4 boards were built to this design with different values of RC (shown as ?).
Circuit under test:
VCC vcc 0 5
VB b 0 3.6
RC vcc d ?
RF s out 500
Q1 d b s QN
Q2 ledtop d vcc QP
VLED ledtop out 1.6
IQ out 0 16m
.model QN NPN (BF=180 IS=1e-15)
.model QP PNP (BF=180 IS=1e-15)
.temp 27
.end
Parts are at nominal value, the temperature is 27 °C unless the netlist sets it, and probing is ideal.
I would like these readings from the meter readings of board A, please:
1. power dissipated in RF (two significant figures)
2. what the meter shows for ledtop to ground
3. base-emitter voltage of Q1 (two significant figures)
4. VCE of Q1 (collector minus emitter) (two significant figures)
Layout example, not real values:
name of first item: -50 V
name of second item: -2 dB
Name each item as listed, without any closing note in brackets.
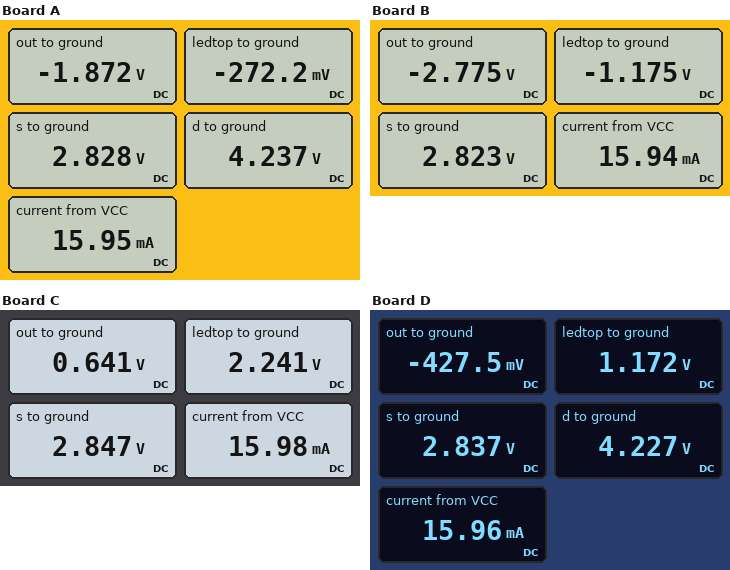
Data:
power dissipated in RF: 44 mW
what the meter shows for ledtop to ground: -272.2 mV
base-emitter voltage of Q1: 770 mV
VCE of Q1 (collector minus emitter): 1.4 V
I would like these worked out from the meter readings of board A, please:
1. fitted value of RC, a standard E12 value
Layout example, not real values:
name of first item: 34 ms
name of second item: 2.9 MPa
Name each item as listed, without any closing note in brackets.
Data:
fitted value of RC, a standard E12 value: 82 Ω
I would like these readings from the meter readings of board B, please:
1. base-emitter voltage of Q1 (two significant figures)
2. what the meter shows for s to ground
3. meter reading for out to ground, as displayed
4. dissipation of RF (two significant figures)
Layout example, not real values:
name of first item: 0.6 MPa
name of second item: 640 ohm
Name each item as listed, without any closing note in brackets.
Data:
base-emitter voltage of Q1: 780 mV
what the meter shows for s to ground: 2.823 V
meter reading for out to ground, as displayed: -2.775 V
dissipation of RF: 63 mW
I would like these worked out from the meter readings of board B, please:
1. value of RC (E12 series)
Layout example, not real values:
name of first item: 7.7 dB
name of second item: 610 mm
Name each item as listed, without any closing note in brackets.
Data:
value of RC: 68 Ω
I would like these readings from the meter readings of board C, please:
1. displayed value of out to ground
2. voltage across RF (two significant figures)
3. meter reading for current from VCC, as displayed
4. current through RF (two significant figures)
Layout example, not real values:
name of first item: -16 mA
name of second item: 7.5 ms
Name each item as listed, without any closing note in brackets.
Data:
displayed value of out to ground: 0.641 V
voltage across RF: 2.2 V
meter reading for current from VCC, as displayed: 15.98 mA
current through RF: 4.4 mA
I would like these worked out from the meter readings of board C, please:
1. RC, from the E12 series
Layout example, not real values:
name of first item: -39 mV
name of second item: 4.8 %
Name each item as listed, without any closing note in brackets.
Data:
RC, from the E12 series: 180 Ω
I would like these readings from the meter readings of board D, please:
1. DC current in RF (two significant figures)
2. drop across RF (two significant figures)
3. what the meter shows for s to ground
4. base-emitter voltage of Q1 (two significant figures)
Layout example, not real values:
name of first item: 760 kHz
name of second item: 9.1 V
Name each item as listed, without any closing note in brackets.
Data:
DC current in RF: 6.5 mA
drop across RF: 3.3 V
what the meter shows for s to ground: 2.837 V
base-emitter voltage of Q1: 760 mV
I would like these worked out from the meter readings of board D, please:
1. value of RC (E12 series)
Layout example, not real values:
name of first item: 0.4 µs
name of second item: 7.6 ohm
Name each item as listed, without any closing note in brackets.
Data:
value of RC: 120 Ω
